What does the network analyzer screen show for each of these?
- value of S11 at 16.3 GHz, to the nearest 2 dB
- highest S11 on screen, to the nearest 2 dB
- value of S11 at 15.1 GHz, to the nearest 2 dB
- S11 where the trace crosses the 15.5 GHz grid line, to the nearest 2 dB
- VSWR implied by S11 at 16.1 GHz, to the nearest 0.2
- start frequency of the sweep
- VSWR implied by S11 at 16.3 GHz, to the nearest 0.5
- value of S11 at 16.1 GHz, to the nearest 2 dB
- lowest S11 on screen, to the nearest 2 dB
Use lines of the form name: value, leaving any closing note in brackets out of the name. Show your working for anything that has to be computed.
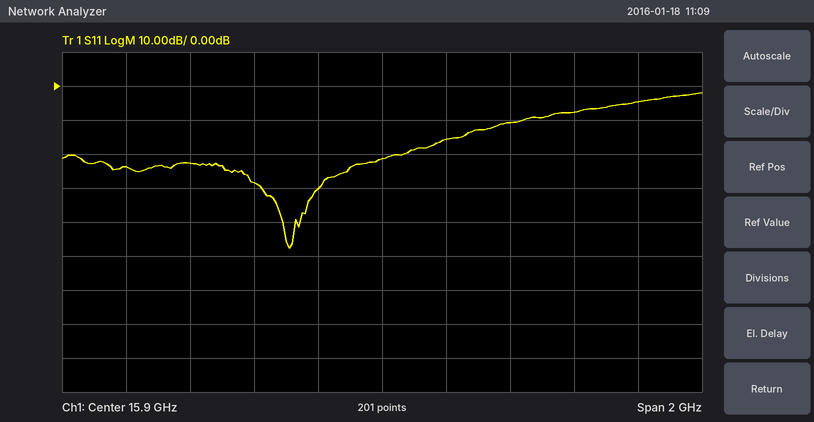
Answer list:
value of S11 at 16.3 GHz, to the nearest 2 dB: -10 dB
highest S11 on screen, to the nearest 2 dB: -2 dB
value of S11 at 15.1 GHz, to the nearest 2 dB: -24 dB
S11 where the trace crosses the 15.5 GHz grid line, to the nearest 2 dB: -28 dB
VSWR implied by S11 at 16.1 GHz, to the nearest 0.2: |Γ| = 10^(-16/20) = 0.1585; VSWR = (1 + 0.1585)/(1 − 0.1585) ≈ 1.4
start frequency of the sweep: 14.9 GHz
VSWR implied by S11 at 16.3 GHz, to the nearest 0.5: |Γ| = 10^(-10/20) = 0.3162; VSWR = (1 + 0.3162)/(1 − 0.3162) ≈ 1.92, so 2.0 to the nearest 0.5
value of S11 at 16.1 GHz, to the nearest 2 dB: -16 dB
lowest S11 on screen, to the nearest 2 dB: -48 dB
